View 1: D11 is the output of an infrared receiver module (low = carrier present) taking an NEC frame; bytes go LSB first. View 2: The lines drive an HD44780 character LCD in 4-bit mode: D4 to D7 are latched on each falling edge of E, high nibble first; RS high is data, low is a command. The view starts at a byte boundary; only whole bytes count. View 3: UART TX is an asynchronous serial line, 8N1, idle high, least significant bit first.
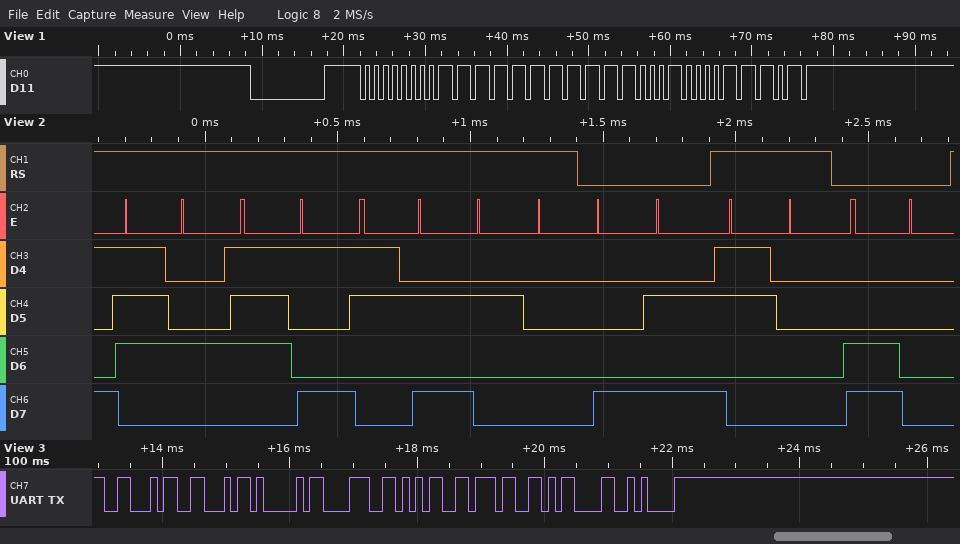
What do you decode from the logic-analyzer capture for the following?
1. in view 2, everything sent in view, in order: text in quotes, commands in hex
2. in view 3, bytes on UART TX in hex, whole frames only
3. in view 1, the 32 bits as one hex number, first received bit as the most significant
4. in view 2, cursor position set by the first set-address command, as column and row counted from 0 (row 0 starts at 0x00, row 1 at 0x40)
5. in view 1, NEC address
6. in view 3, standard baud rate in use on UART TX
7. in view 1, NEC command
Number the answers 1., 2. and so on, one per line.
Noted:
1. "ty: " 0x8A "0" 0xC0
2. 0x46 0x46 0x41 0x38 0x35 0x37 0x0D 0x0A
3. 0x00FFE21D
4. column 10, row 0
5. 0x00
6. 9600 baud
7. 0x47
